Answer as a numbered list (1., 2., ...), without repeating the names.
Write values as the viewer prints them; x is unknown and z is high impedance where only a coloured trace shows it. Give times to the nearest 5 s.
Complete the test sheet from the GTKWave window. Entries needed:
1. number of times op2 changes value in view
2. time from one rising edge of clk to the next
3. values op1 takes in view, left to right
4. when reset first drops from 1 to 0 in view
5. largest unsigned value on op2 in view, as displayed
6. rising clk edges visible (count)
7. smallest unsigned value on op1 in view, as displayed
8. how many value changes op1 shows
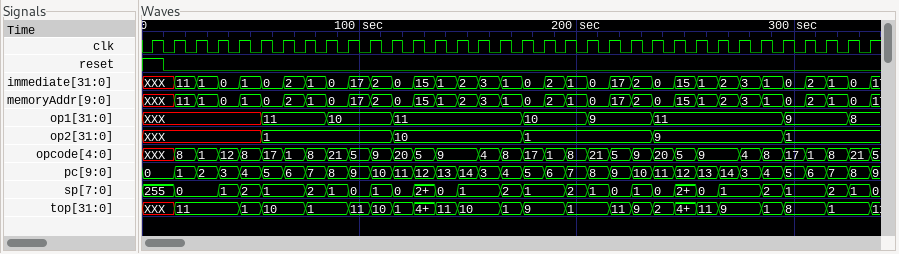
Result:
1. 5
2. 10 s
3. XXX, 11, 10, 11, 10, 9, 11, 9, 8
4. 10 s
5. 10
6. 34
7. 8
8. 8
